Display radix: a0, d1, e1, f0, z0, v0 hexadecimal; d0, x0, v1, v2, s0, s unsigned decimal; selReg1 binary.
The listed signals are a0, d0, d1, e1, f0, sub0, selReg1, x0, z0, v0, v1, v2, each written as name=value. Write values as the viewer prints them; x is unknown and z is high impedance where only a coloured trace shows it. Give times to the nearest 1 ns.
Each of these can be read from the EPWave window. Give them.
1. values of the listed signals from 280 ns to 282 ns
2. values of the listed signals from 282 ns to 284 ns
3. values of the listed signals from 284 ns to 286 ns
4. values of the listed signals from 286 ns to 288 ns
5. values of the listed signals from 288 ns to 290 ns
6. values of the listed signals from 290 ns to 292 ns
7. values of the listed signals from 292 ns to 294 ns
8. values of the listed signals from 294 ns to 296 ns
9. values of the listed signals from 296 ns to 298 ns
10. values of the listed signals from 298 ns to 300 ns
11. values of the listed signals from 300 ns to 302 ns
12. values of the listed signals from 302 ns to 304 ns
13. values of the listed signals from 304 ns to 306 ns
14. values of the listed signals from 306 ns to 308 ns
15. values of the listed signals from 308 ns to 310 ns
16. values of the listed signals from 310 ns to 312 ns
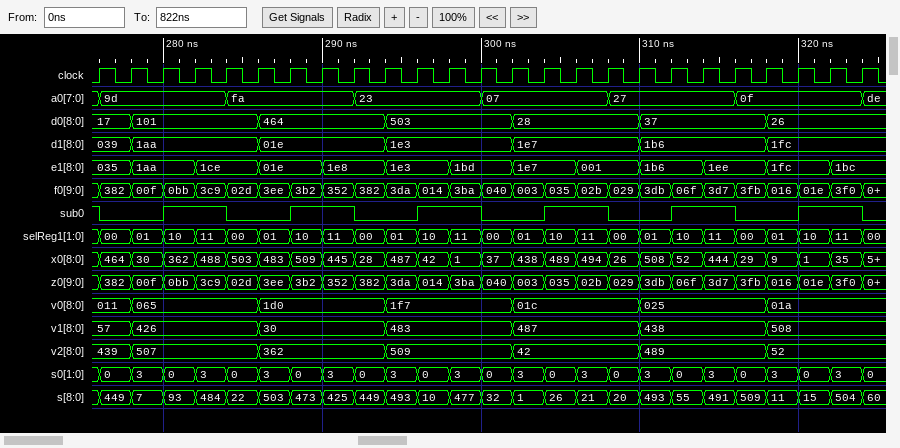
a0=9d, d0=101, d1=1aa, e1=1aa, f0=0bb, sub0=1, selReg1=10, x0=362, z0=0bb, v0=065, v1=426, v2=507
a0=9d, d0=101, d1=1aa, e1=1ce, f0=3c9, sub0=1, selReg1=11, x0=488, z0=3c9, v0=065, v1=426, v2=507
a0=fa, d0=101, d1=1aa, e1=1ce, f0=02d, sub0=0, selReg1=00, x0=503, z0=02d, v0=065, v1=426, v2=507
a0=fa, d0=464, d1=01e, e1=01e, f0=3ee, sub0=0, selReg1=01, x0=483, z0=3ee, v0=1d0, v1=30, v2=362
a0=fa, d0=464, d1=01e, e1=01e, f0=3b2, sub0=1, selReg1=10, x0=509, z0=3b2, v0=1d0, v1=30, v2=362
a0=fa, d0=464, d1=01e, e1=1e8, f0=352, sub0=1, selReg1=11, x0=445, z0=352, v0=1d0, v1=30, v2=362
a0=23, d0=464, d1=01e, e1=1e8, f0=382, sub0=0, selReg1=00, x0=28, z0=382, v0=1d0, v1=30, v2=362
a0=23, d0=503, d1=1e3, e1=1e3, f0=3da, sub0=0, selReg1=01, x0=487, z0=3da, v0=1f7, v1=483, v2=509
a0=23, d0=503, d1=1e3, e1=1e3, f0=014, sub0=1, selReg1=10, x0=42, z0=014, v0=1f7, v1=483, v2=509
a0=23, d0=503, d1=1e3, e1=1bd, f0=3ba, sub0=1, selReg1=11, x0=1, z0=3ba, v0=1f7, v1=483, v2=509
a0=07, d0=503, d1=1e3, e1=1bd, f0=040, sub0=0, selReg1=00, x0=37, z0=040, v0=1f7, v1=483, v2=509
a0=07, d0=28, d1=1e7, e1=1e7, f0=003, sub0=0, selReg1=01, x0=438, z0=003, v0=01c, v1=487, v2=42
a0=07, d0=28, d1=1e7, e1=1e7, f0=035, sub0=1, selReg1=10, x0=489, z0=035, v0=01c, v1=487, v2=42
a0=07, d0=28, d1=1e7, e1=001, f0=02b, sub0=1, selReg1=11, x0=494, z0=02b, v0=01c, v1=487, v2=42
a0=27, d0=28, d1=1e7, e1=001, f0=029, sub0=0, selReg1=00, x0=26, z0=029, v0=01c, v1=487, v2=42
a0=27, d0=37, d1=1b6, e1=1b6, f0=3db, sub0=0, selReg1=01, x0=508, z0=3db, v0=025, v1=438, v2=489
